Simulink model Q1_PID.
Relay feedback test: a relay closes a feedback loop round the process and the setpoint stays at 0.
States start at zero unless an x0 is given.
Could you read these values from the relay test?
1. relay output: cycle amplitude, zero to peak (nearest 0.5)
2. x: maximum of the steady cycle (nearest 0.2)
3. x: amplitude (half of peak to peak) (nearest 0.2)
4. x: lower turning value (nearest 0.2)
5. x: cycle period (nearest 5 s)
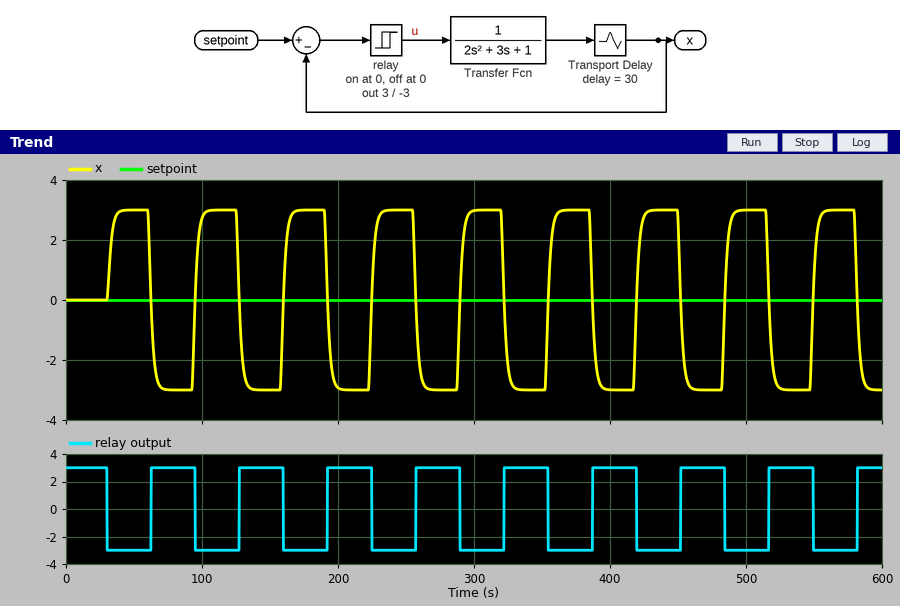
3.0
3.0
3.0
-3.0
65 s
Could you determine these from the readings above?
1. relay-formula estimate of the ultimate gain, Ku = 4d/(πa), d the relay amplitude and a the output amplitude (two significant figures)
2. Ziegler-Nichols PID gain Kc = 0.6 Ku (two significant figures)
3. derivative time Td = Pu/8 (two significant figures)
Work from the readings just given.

1.3
0.78
8.1 s
